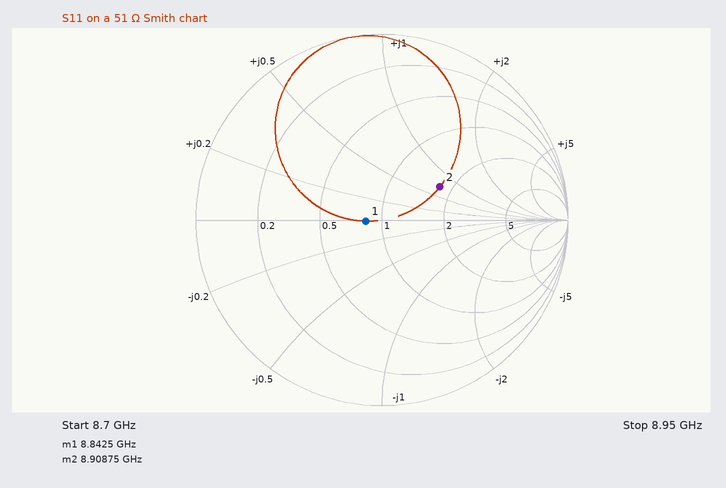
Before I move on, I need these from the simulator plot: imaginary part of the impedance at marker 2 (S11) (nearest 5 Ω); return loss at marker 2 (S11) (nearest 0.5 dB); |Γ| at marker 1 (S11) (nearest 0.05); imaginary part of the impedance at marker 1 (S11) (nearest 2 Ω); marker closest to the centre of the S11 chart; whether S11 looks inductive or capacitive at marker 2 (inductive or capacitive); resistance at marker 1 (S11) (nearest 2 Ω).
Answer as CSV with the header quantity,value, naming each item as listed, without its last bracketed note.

quantity,value
imaginary part of the impedance at marker 2 (S11),+35 Ω
return loss at marker 2 (S11),9.0 dB
|Γ| at marker 1 (S11),0.10
imaginary part of the impedance at marker 1 (S11),0 Ω
marker closest to the centre of the S11 chart,marker 1
whether S11 looks inductive or capacitive at marker 2,inductive
resistance at marker 1 (S11),42 Ω
